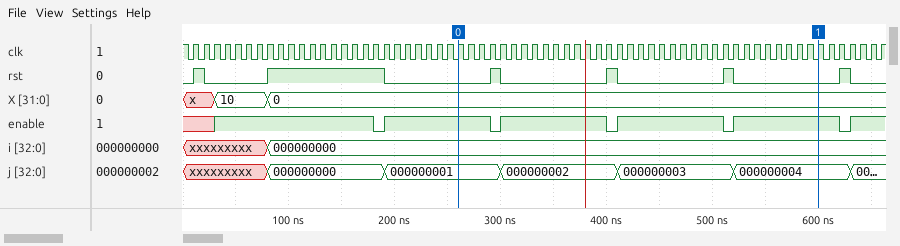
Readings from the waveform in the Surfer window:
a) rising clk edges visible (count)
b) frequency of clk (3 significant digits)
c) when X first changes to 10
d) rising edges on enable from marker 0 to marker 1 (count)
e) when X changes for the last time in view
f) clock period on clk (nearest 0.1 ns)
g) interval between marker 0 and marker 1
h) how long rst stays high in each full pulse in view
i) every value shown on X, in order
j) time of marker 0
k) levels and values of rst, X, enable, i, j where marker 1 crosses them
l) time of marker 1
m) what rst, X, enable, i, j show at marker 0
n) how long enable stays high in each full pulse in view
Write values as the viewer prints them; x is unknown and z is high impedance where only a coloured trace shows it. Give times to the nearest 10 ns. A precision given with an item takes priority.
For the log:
66
100 MHz
30 ns
3
80 ns
10 ns
340 ns
10 ns, 110 ns, 10 ns, 10 ns, 10 ns, 10 ns
x, 10, 0
260 ns
rst=0, X=0, enable=1, i=000000000, j=000000004
600 ns
rst=0, X=0, enable=1, i=000000000, j=000000001
100 ns, 100 ns, 100 ns, 100 ns
